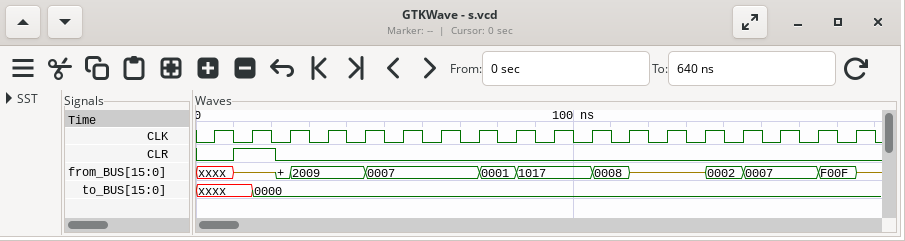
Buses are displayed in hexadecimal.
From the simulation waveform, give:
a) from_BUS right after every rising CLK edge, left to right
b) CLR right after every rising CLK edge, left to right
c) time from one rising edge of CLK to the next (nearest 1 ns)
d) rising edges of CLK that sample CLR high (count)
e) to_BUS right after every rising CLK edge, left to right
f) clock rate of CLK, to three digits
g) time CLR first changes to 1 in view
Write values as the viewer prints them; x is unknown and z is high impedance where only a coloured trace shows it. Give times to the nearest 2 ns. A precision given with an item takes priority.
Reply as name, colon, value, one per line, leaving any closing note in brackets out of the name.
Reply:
from_BUS right after every rising CLK edge, left to right: xxxx, z, 2009, 2009, 0007, 0007, 0007, 0001, 1017, 1017, 0008, z, z, 0002, 0007, 0007, F00F, z
CLR right after every rising CLK edge, left to right: 0 1 0 0 0 0 0 0 0 0 0 0 0 0 0 0 0 0
time from one rising edge of CLK to the next: 10 ns
rising edges of CLK that sample CLR high: 1
to_BUS right after every rising CLK edge, left to right: xxxx, 0000, 0000, 0000, 0000, 0000, 0000, 0000, 0000, 0000, 0000, 0000, 0000, 0000, 0000, 0000, 0000, 0000
clock rate of CLK, to three digits: 100 MHz
time CLR first changes to 1 in view: 10 ns
